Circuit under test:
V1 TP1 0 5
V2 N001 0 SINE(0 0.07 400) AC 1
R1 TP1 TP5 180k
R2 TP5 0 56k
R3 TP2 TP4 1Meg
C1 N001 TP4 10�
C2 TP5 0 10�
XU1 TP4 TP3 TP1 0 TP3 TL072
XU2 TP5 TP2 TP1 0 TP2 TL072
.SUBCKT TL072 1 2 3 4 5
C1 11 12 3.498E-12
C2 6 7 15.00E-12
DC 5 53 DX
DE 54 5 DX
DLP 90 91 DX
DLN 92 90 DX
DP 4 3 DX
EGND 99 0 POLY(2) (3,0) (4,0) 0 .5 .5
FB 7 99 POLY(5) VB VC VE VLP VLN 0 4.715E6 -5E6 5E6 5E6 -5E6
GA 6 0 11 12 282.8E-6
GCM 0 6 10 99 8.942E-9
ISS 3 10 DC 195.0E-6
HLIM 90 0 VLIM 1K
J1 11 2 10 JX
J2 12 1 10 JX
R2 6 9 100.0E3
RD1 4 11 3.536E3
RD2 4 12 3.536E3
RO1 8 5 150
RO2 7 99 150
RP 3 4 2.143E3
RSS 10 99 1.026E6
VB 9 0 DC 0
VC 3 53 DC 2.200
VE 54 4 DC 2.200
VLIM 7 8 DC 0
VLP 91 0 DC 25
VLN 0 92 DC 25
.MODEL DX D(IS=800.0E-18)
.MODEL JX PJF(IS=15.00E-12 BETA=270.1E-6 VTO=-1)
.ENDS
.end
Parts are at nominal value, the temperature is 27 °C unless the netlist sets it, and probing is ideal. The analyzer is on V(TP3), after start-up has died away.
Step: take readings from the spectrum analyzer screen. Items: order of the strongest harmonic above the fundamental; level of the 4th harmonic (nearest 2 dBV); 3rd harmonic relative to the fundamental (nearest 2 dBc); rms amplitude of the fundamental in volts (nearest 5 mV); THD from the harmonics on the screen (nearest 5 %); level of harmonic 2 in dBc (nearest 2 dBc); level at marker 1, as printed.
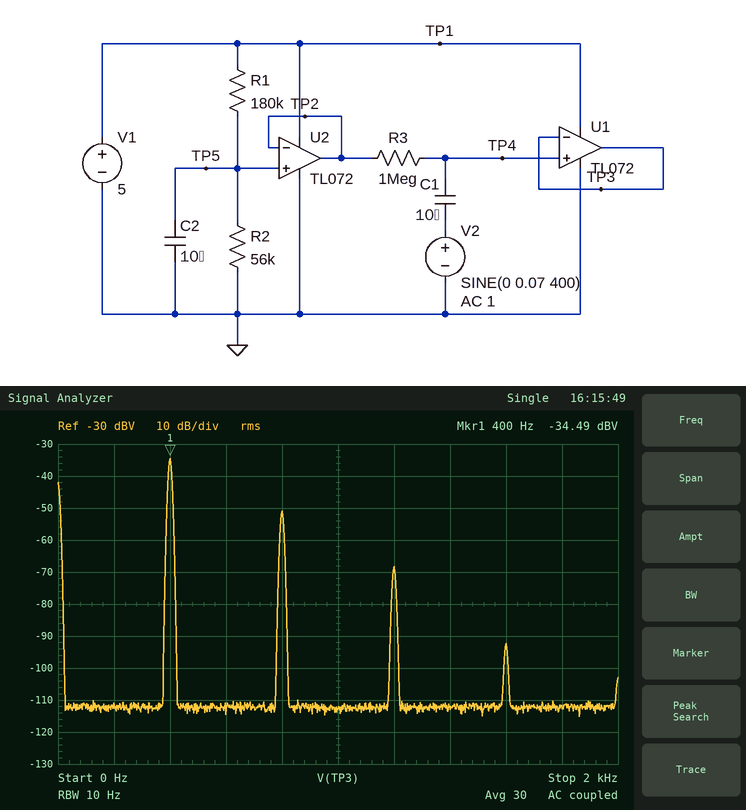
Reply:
2
-92 dBV
-34 dBc
20 mV
15 %
-16 dBc
-34.49 dBV
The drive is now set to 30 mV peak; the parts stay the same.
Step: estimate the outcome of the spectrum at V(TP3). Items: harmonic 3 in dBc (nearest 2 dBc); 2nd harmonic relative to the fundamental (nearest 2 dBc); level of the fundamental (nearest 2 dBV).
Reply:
-48 dBc
-24 dBc
-42 dBV
